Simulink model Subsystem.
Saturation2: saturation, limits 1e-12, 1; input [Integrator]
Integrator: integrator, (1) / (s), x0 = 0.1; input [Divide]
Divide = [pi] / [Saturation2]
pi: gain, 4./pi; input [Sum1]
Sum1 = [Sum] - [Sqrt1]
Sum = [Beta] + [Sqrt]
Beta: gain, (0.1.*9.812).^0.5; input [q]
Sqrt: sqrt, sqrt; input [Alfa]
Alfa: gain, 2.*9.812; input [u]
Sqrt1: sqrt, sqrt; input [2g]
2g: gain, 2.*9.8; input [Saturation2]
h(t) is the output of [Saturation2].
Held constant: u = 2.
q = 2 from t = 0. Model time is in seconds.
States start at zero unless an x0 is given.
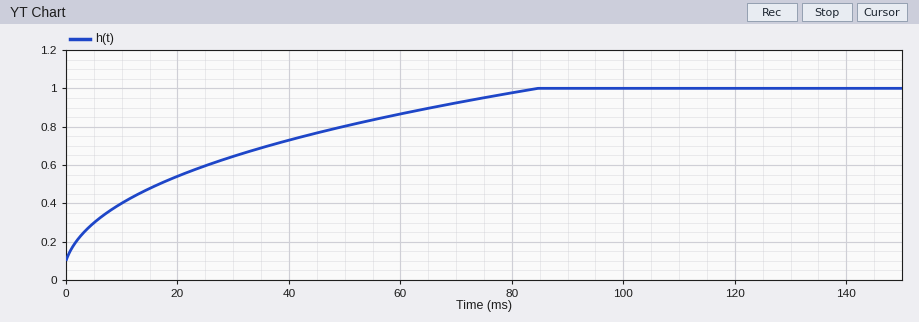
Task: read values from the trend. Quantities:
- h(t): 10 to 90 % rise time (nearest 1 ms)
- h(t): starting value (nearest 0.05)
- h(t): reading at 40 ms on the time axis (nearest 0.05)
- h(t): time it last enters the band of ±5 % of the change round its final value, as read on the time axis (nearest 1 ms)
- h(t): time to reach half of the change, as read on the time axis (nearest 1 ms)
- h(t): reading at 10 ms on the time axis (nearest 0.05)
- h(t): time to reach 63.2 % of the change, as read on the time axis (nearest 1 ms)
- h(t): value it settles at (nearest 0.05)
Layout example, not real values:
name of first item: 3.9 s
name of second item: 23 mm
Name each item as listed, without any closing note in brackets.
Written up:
h(t): 10 to 90 % rise time: 66 ms
h(t): starting value: 0.10
h(t): reading at 40 ms on the time axis: 0.75
h(t): time it last enters the band of ±5 % of the change round its final value, as read on the time axis: 76 ms
h(t): time to reach half of the change, as read on the time axis: 21 ms
h(t): reading at 10 ms on the time axis: 0.40
h(t): time to reach 63.2 % of the change, as read on the time axis: 33 ms
h(t): value it settles at: 1.00
